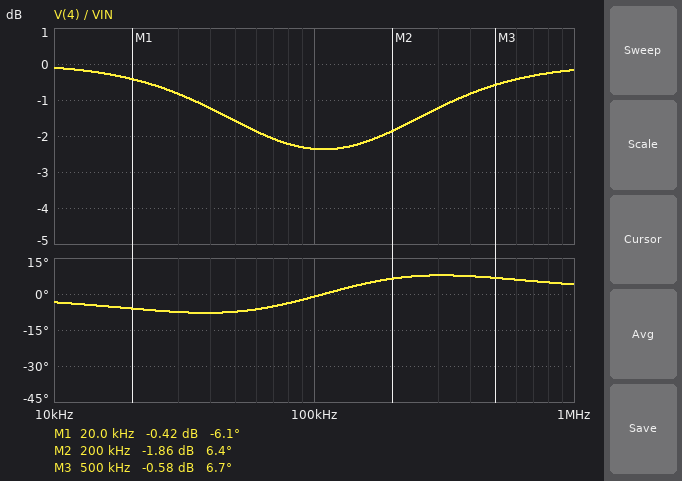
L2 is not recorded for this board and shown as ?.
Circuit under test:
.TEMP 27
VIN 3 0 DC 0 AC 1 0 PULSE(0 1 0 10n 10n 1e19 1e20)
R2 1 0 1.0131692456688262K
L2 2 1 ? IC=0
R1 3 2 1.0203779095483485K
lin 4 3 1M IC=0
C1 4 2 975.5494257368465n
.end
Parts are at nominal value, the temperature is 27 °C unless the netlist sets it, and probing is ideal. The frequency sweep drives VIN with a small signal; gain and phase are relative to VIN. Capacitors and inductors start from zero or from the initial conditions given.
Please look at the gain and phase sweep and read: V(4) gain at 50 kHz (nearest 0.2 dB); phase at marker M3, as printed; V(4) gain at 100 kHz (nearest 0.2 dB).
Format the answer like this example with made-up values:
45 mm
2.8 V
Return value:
-1.6 dB
6.7 deg
-2.4 dB
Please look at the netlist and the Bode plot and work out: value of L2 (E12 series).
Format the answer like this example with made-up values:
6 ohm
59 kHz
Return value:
2.2 mH
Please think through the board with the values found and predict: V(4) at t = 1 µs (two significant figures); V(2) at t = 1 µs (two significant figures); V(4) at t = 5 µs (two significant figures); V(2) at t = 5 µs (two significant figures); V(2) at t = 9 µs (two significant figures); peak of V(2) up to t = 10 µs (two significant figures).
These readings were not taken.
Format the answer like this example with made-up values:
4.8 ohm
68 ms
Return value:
810 mV
810 mV
920 mV
920 mV
970 mV
1.0 V
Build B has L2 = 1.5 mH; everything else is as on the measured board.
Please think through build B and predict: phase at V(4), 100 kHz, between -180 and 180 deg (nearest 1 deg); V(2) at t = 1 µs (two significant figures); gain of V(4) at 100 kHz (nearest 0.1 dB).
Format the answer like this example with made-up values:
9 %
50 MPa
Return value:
-4 deg
770 mV
-2.8 dB
